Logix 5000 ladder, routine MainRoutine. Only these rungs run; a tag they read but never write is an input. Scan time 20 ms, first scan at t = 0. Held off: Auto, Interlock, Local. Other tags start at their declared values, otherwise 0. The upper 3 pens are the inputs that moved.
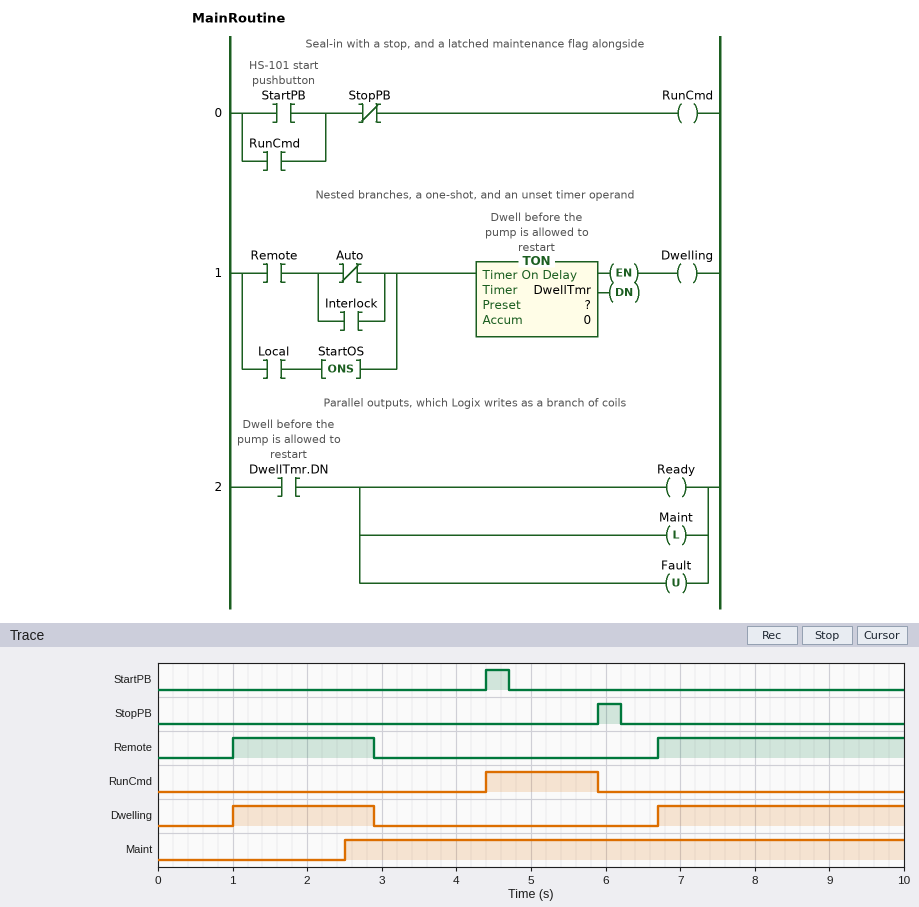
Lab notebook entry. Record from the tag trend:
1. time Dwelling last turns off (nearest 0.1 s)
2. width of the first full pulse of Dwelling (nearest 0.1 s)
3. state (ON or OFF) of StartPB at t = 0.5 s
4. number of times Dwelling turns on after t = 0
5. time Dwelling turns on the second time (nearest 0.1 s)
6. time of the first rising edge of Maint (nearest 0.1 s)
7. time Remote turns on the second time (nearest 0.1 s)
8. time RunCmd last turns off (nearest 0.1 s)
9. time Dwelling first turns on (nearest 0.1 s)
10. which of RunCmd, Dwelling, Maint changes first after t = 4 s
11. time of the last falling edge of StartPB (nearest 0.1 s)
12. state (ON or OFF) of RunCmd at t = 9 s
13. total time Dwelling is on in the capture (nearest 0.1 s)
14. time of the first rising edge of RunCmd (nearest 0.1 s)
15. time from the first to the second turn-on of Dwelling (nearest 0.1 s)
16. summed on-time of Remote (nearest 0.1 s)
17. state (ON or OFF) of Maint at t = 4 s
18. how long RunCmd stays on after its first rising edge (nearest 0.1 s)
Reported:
2.9 s
1.9 s
OFF
2
6.7 s
2.5 s
6.7 s
5.9 s
1.0 s
RunCmd
4.7 s
OFF
5.2 s
4.4 s
5.7 s
5.2 s
ON
1.5 s
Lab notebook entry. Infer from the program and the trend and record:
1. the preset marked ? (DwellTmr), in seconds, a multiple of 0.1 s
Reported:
1.5 s
